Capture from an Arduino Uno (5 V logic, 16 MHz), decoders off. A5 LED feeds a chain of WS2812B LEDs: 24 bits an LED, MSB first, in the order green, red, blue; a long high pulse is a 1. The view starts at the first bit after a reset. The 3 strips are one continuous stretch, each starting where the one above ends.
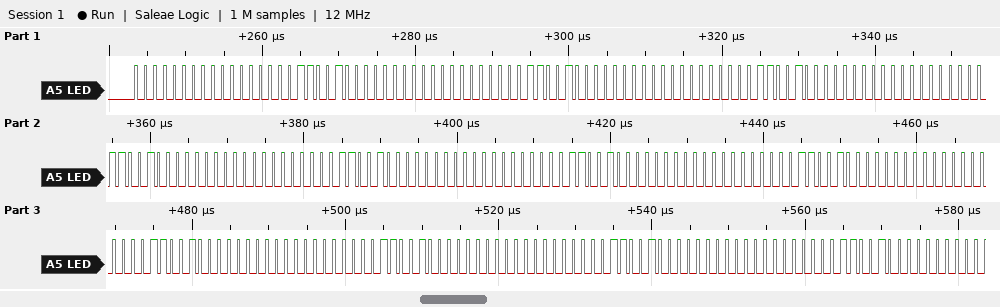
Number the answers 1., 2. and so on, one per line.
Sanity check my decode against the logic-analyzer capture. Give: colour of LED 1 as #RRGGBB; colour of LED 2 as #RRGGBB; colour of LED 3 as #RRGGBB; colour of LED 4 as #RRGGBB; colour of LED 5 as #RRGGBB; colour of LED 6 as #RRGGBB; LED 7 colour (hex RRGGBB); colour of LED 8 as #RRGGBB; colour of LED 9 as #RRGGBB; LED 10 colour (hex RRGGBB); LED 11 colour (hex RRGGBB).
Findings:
1. #000064
2. #000064
3. #000064
4. #000064
5. #000064
6. #000064
7. #000064
8. #000064
9. #000064
10. #000064
11. #000064
